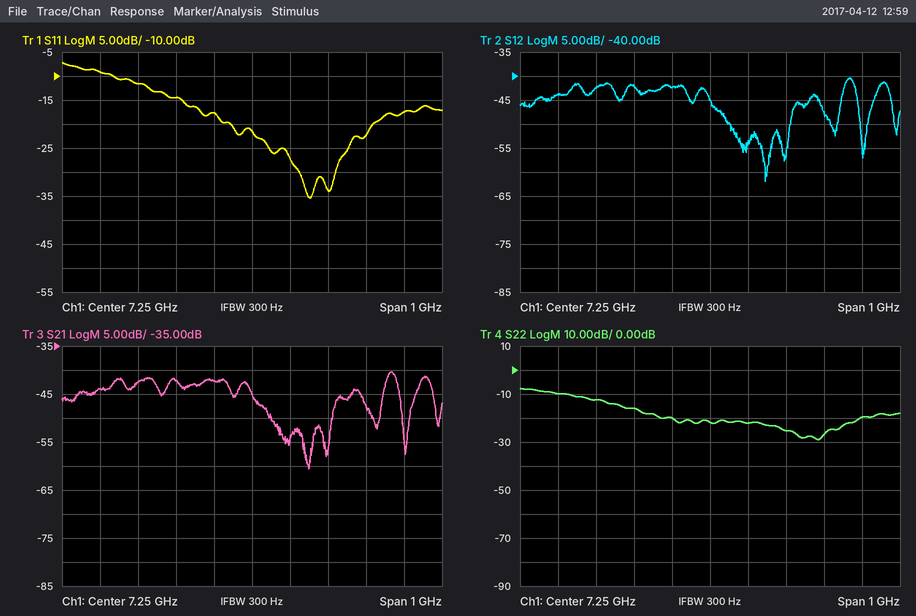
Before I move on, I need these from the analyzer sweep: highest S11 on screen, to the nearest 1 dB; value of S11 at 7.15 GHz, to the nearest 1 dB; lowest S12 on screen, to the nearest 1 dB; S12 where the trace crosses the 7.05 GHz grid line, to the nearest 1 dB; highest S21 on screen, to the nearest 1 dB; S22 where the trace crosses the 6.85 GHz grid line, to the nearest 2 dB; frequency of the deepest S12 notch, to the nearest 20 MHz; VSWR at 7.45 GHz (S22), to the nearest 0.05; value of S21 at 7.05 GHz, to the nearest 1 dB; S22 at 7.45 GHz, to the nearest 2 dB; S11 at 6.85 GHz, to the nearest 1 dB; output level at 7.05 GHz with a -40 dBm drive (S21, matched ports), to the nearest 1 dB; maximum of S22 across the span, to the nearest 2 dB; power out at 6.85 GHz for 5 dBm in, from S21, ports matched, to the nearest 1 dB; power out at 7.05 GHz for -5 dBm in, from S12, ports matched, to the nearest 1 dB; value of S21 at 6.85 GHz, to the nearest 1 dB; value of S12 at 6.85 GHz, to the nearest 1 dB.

-7 dB
-18 dB
-62 dB
-42 dB
-40 dB
-10 dB
7.40 GHz
1.10
-42 dB
-26 dB
-9 dB
-82 dBm
-8 dB
-39 dBm
-47 dBm
-44 dB
-44 dB
